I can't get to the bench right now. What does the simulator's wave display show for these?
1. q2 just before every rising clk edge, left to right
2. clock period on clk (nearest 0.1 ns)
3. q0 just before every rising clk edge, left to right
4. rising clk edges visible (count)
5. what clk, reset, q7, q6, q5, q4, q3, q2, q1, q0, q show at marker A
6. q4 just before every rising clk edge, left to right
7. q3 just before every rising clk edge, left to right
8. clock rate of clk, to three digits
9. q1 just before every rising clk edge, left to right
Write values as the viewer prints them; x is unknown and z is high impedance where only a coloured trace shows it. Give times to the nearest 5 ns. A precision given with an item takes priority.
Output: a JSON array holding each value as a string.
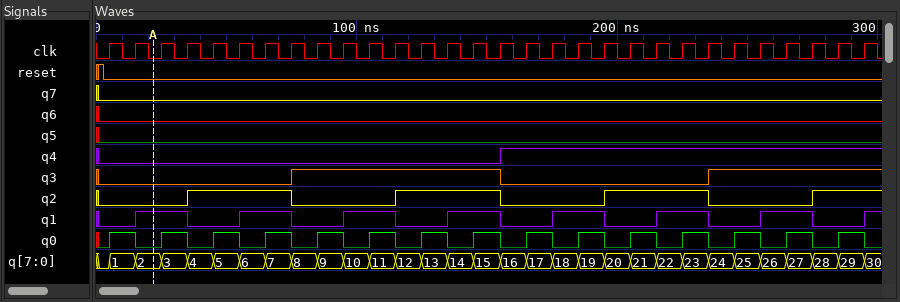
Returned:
["0 0 0 0 1 1 1 1 0 0 0 0 1 1 1 1 0 0 0 0 1 1 1 1 0 0 0 0 1 1", "10 ns", "0 1 0 1 0 1 0 1 0 1 0 1 0 1 0 1 0 1 0 1 0 1 0 1 0 1 0 1 0 1", "30", "clk=0, reset=0, q7=0, q6=0, q5=0, q4=0, q3=0, q2=0, q1=1, q0=0, q=2", "0 0 0 0 0 0 0 0 0 0 0 0 0 0 0 0 1 1 1 1 1 1 1 1 1 1 1 1 1 1", "0 0 0 0 0 0 0 0 1 1 1 1 1 1 1 1 0 0 0 0 0 0 0 0 1 1 1 1 1 1", "100 MHz", "0 0 1 1 0 0 1 1 0 0 1 1 0 0 1 1 0 0 1 1 0 0 1 1 0 0 1 1 0 0"]
